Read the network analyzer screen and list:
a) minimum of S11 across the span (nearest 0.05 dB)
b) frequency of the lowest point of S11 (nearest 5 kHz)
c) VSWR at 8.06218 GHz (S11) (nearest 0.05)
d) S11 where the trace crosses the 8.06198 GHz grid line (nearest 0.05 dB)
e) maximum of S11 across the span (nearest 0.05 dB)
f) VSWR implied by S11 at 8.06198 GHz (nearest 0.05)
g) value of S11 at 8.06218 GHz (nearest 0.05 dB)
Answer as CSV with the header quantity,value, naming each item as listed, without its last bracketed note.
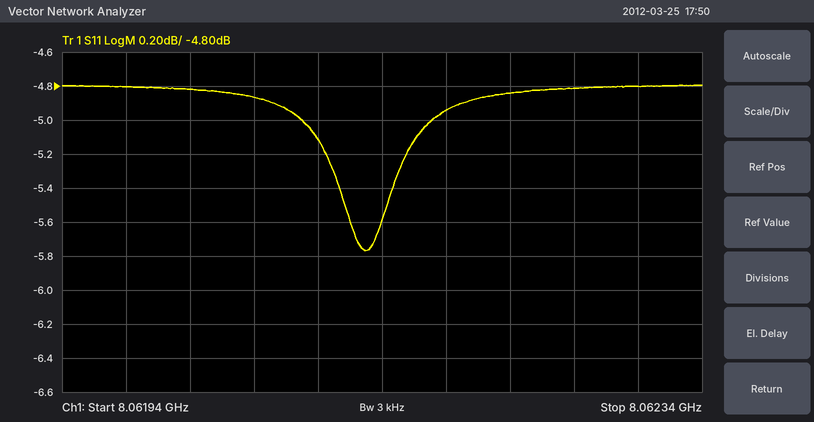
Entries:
quantity,value
minimum of S11 across the span,-5.75 dB
frequency of the lowest point of S11,8.062130 GHz
VSWR at 8.06218 GHz (S11),3.60
S11 where the trace crosses the 8.06198 GHz grid line,-4.80 dB
maximum of S11 across the span,-4.80 dB
VSWR implied by S11 at 8.06198 GHz,3.70
value of S11 at 8.06218 GHz,-4.95 dB
